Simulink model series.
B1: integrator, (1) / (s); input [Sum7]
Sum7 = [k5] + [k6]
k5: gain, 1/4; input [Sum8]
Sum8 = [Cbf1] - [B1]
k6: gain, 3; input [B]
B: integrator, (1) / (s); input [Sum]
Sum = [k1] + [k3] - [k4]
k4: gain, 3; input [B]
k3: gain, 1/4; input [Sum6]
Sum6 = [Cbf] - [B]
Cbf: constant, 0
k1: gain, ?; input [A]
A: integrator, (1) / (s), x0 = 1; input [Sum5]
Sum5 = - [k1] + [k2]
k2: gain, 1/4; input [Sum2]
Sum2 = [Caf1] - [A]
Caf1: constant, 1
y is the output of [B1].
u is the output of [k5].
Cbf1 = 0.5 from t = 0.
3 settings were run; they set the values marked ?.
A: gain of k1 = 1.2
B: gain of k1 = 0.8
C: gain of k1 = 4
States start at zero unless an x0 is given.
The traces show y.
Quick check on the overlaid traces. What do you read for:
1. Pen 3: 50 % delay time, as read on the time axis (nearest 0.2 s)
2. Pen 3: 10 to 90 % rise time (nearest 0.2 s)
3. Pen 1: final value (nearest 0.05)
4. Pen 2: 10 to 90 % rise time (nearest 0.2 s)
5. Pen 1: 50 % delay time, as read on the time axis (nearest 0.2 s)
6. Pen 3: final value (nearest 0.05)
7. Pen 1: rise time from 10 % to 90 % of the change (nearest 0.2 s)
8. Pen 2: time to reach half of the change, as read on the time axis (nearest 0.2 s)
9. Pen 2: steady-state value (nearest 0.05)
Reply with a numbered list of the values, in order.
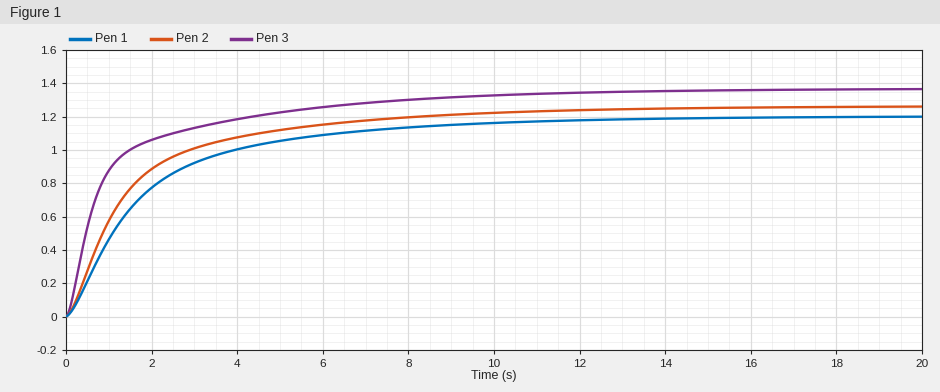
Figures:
1. 0.6 s
2. 5.0 s
3. 1.20
4. 5.2 s
5. 1.4 s
6. 1.35
7. 5.4 s
8. 1.2 s
9. 1.25
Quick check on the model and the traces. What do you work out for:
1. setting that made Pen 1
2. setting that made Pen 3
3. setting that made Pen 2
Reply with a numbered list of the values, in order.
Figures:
1. B
2. C
3. A
